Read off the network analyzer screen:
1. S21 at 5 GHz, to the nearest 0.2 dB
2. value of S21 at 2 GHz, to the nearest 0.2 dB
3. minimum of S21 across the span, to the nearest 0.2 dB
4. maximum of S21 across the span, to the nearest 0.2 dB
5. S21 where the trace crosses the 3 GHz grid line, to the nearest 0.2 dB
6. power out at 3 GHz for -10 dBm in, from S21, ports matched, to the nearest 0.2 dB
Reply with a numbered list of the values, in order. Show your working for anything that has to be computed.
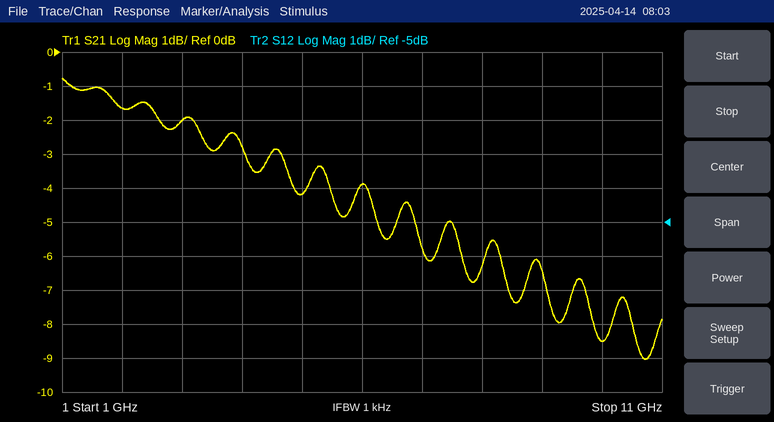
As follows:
1. -4.2 dB
2. -1.6 dB
3. -9.0 dB
4. -0.8 dB
5. -2.0 dB
6. -10 dBm + (-2.0 dB) = -12.0 dBm
